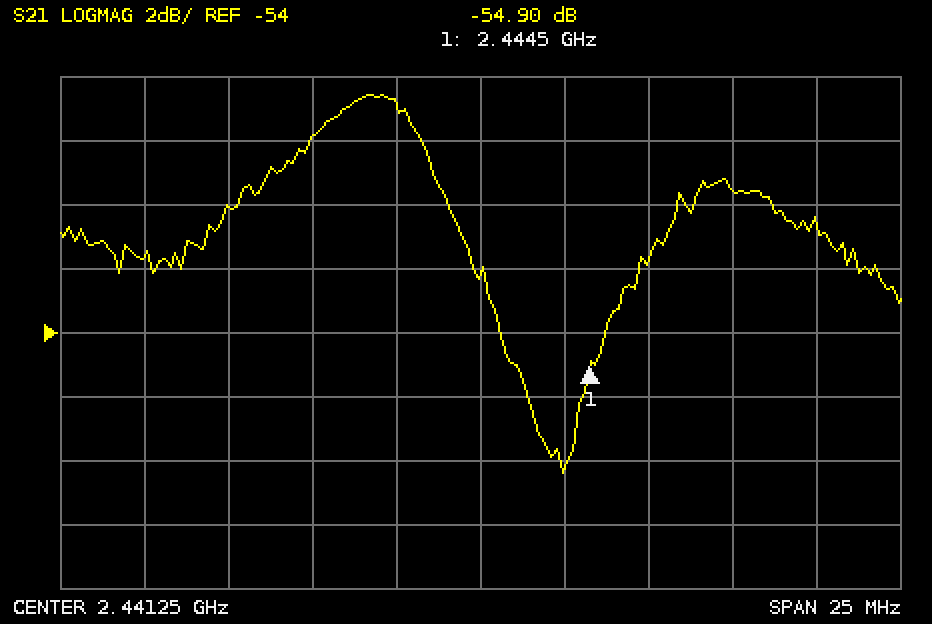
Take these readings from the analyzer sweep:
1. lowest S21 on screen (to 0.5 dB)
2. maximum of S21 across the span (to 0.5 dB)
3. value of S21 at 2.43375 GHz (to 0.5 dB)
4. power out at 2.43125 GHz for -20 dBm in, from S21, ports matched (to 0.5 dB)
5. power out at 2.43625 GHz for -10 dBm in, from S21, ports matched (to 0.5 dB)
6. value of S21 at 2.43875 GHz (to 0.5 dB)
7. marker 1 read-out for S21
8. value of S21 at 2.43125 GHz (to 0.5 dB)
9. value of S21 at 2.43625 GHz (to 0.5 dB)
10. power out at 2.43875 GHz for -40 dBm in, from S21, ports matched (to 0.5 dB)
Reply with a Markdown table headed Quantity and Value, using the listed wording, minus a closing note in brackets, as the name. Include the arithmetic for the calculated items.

| Quantity | Value |
|---|---|
| lowest S21 on screen | -58.5 dB |
| maximum of S21 across the span | -46.5 dB |
| value of S21 at 2.43375 GHz | -50.0 dB |
| power out at 2.43125 GHz for -20 dBm in, from S21, ports matched | -20 dBm + (-51.5 dB) = -71.5 dBm |
| power out at 2.43625 GHz for -10 dBm in, from S21, ports matched | -10 dBm + (-48.0 dB) = -58.0 dBm |
| value of S21 at 2.43875 GHz | -47.0 dB |
| marker 1 read-out for S21 | -54.90 dB |
| value of S21 at 2.43125 GHz | -51.5 dB |
| value of S21 at 2.43625 GHz | -48.0 dB |
| power out at 2.43875 GHz for -40 dBm in, from S21, ports matched | -40 dBm + (-47.0 dB) = -87.0 dBm |
